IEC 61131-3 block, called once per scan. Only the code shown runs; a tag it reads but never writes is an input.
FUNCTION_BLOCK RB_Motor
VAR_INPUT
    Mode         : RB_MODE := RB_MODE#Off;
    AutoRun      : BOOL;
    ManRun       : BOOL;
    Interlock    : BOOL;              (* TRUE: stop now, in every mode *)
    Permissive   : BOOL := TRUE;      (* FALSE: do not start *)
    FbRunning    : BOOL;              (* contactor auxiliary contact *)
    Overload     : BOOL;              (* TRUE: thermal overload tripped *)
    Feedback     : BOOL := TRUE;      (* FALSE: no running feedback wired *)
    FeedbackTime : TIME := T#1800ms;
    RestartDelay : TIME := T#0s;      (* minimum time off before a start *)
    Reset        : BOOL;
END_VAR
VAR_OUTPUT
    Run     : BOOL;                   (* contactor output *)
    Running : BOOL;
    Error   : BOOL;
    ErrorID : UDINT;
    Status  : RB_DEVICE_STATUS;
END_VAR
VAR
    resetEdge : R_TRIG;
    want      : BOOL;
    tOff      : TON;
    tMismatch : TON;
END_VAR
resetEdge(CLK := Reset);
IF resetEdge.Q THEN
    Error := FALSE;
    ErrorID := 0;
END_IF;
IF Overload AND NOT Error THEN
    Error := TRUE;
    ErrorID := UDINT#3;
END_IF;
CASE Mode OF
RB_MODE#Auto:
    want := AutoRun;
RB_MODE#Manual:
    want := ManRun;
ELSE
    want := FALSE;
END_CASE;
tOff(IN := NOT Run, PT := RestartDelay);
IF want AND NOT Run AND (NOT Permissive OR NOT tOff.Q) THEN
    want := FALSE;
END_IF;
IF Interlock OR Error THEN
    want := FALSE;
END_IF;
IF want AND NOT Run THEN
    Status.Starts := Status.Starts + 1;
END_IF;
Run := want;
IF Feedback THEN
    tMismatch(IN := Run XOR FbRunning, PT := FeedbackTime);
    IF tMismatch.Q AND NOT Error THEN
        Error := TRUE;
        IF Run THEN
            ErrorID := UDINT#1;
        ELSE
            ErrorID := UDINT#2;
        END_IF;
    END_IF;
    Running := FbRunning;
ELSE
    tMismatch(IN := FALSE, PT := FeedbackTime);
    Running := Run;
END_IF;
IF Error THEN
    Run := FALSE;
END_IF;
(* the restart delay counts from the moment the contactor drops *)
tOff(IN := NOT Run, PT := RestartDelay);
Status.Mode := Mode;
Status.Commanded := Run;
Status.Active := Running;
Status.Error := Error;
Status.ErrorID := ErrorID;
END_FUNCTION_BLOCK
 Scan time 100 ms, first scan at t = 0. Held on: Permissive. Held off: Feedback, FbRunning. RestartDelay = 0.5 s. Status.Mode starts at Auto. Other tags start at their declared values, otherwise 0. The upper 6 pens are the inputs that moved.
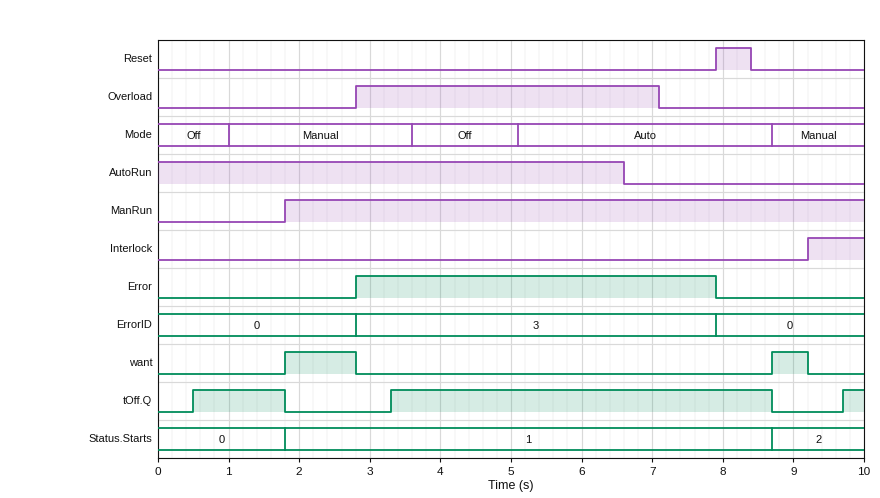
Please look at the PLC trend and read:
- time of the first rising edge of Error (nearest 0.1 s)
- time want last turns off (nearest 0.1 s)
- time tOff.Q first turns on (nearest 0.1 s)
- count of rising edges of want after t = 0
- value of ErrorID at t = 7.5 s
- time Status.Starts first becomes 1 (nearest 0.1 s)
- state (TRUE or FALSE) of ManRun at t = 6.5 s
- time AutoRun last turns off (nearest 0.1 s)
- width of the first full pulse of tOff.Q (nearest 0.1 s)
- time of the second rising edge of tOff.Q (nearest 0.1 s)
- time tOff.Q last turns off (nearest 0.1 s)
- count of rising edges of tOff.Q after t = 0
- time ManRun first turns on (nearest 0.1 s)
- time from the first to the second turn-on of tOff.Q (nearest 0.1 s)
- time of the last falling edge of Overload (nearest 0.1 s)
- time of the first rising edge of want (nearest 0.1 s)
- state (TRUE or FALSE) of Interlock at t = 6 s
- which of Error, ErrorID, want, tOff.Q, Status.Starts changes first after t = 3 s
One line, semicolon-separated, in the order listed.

2.8 s; 9.2 s; 0.5 s; 2; 3; 1.8 s; TRUE; 6.6 s; 1.3 s; 3.3 s; 8.7 s; 3; 1.8 s; 2.8 s; 7.1 s; 1.8 s; FALSE; tOff.Q
